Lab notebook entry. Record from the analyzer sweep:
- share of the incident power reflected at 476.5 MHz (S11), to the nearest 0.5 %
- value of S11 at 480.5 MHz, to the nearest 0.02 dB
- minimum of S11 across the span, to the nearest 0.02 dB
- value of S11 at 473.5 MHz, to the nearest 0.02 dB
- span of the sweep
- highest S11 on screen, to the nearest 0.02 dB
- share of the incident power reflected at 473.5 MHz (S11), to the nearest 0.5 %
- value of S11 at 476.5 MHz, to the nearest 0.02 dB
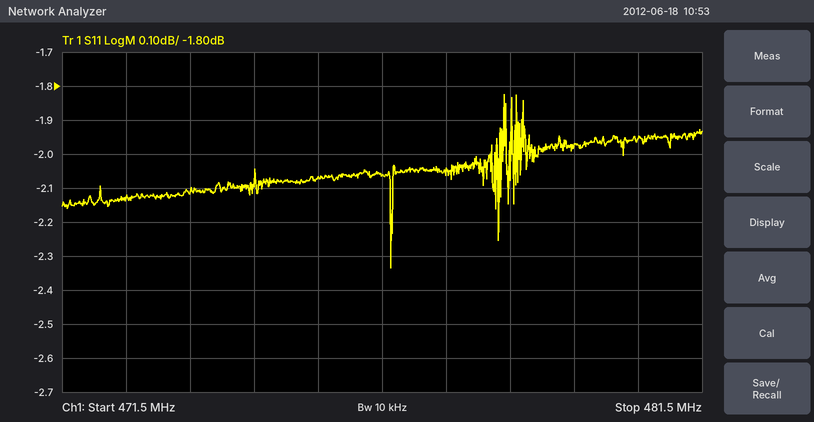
62.0 %
-1.96 dB
-2.34 dB
-2.12 dB
10 MHz
-1.82 dB
61.5 %
-2.06 dB
